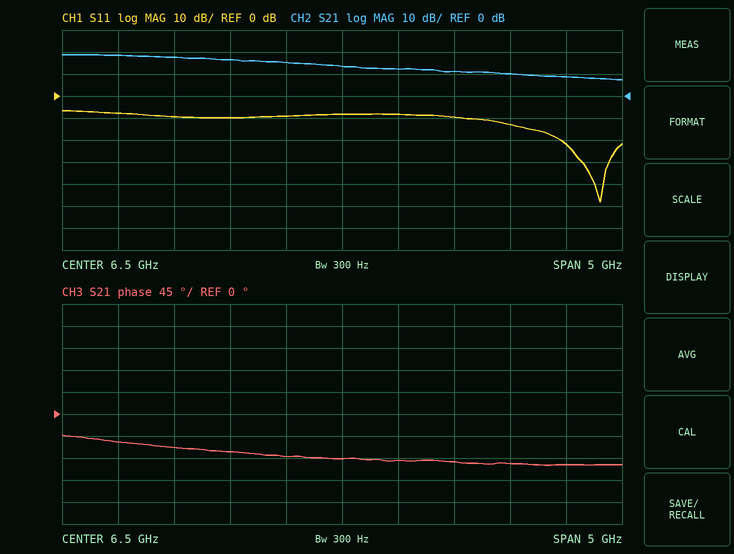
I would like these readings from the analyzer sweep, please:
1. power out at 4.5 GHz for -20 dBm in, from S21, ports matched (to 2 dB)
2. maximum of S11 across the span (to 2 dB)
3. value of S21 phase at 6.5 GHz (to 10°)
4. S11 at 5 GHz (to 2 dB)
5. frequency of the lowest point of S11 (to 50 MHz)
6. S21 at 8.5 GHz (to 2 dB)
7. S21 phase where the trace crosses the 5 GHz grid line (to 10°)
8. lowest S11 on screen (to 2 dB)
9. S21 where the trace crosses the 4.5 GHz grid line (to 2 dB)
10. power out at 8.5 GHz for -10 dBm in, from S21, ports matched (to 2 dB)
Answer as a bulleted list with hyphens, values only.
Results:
- -2 dBm
- -6 dB
- -90°
- -10 dB
- 8.80 GHz
- 8 dB
- -70°
- -48 dB
- 18 dB
- -2 dBm
